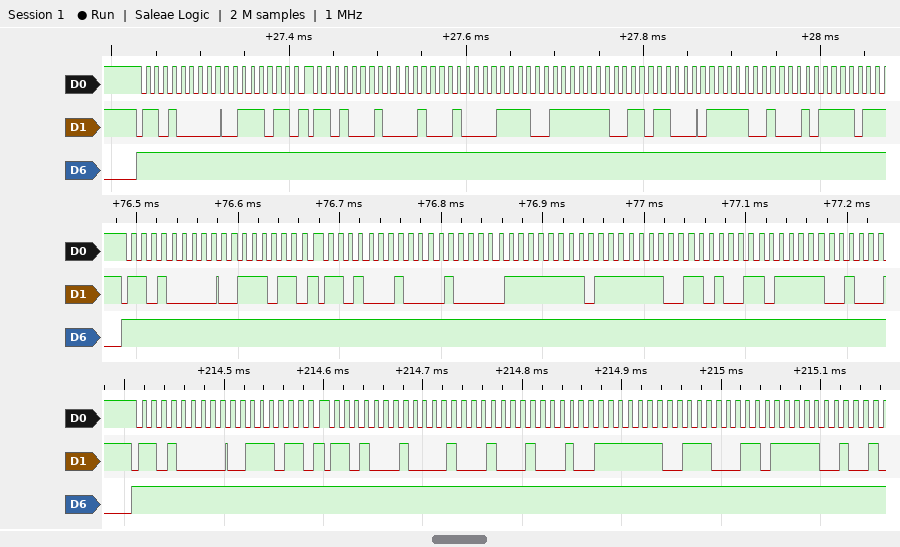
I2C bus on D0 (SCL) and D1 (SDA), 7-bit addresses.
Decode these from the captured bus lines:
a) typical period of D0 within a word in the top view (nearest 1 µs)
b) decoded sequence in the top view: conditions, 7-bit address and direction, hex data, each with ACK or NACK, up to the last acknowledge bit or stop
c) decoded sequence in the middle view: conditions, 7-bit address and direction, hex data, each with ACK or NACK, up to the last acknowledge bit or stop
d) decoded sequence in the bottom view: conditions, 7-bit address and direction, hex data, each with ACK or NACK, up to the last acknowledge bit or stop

10 µs
start, address 68 write ACK, 3B ACK, repeated start, address 68 read ACK, 11 ACK, 1E ACK, FE ACK, D8 ACK, F9 ACK, 2F ACK
start, address 68 write ACK, 3B ACK, repeated start, address 68 read ACK, 10 ACK, FF ACK, FE ACK, D3 ACK, F9 ACK
start, address 68 write ACK, 3B ACK, repeated start, address 68 read ACK, 11 ACK, 22 ACK, FE ACK, E3 ACK, F9 ACK
